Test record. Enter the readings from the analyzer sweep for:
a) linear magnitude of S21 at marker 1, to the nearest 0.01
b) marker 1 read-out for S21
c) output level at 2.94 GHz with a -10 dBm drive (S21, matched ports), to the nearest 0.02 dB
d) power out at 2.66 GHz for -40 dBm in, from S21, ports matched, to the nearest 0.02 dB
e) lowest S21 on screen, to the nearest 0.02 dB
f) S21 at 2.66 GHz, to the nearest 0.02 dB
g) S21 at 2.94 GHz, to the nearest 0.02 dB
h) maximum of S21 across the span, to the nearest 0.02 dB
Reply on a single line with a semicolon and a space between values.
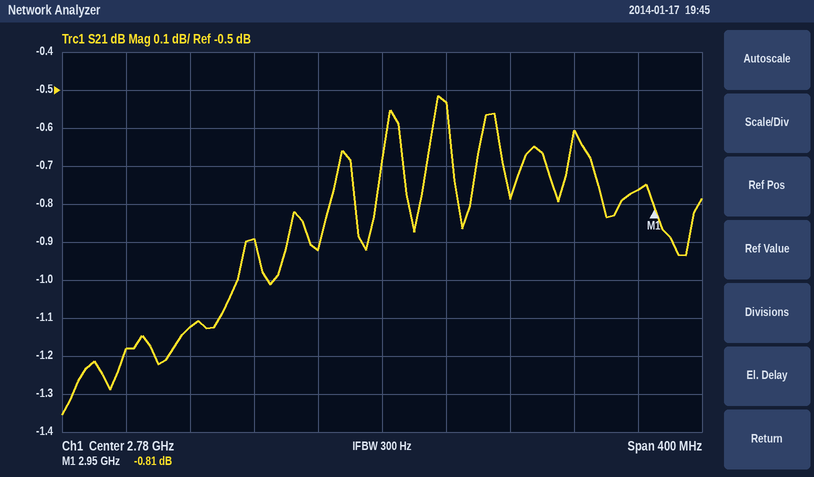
0.91; -0.81 dB; -10.76 dBm; -41.12 dBm; -1.36 dB; -1.12 dB; -0.76 dB; -0.52 dB
